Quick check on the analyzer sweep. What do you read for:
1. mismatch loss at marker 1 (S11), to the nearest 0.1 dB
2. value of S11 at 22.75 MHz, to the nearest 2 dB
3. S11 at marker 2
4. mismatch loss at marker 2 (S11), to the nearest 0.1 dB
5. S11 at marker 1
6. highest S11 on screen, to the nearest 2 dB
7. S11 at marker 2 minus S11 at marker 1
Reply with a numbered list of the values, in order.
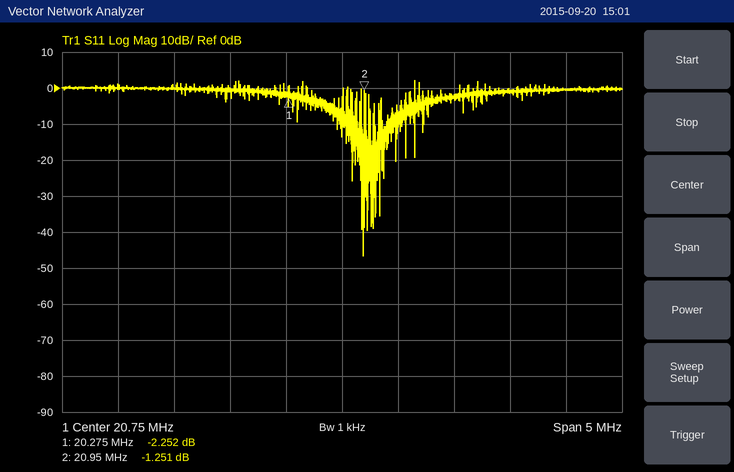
1. 3.9 dB
2. 0 dB
3. -1.251 dB
4. 6.0 dB
5. -2.252 dB
6. 2 dB
7. 1.001 dB
